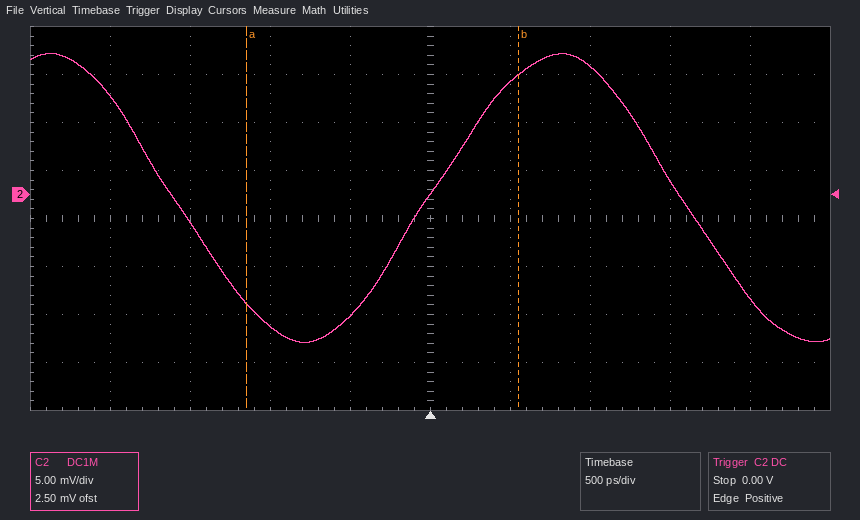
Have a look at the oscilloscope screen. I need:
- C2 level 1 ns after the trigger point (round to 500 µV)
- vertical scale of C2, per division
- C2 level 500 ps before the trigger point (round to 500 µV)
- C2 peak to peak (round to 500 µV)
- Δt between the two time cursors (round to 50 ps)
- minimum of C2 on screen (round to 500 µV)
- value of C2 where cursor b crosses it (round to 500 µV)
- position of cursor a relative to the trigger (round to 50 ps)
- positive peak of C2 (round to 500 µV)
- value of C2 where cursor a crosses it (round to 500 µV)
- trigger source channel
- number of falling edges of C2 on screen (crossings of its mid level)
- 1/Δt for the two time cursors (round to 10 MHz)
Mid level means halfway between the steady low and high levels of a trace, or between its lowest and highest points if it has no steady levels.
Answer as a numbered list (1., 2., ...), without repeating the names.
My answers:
1. 13.5 mV
2. 5 mV
3. -12.5 mV
4. 30.0 mV
5. 1.70 ns
6. -15.5 mV
7. 12.5 mV
8. -1.15 ns
9. 14.5 mV
10. -11.5 mV
11. C2
12. 2
13. 590 MHz
